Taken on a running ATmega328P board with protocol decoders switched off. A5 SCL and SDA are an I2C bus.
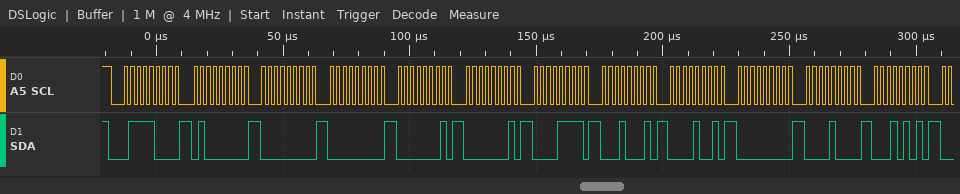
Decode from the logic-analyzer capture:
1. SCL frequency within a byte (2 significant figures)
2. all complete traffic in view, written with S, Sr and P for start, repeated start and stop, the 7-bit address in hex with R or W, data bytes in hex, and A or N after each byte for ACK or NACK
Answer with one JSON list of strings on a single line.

["400 kHz", "S 3CW A 40 A 00 A 00 A 01 A 01 A 0F A 11 A 09 A 00 A 08 A 15 A"]
